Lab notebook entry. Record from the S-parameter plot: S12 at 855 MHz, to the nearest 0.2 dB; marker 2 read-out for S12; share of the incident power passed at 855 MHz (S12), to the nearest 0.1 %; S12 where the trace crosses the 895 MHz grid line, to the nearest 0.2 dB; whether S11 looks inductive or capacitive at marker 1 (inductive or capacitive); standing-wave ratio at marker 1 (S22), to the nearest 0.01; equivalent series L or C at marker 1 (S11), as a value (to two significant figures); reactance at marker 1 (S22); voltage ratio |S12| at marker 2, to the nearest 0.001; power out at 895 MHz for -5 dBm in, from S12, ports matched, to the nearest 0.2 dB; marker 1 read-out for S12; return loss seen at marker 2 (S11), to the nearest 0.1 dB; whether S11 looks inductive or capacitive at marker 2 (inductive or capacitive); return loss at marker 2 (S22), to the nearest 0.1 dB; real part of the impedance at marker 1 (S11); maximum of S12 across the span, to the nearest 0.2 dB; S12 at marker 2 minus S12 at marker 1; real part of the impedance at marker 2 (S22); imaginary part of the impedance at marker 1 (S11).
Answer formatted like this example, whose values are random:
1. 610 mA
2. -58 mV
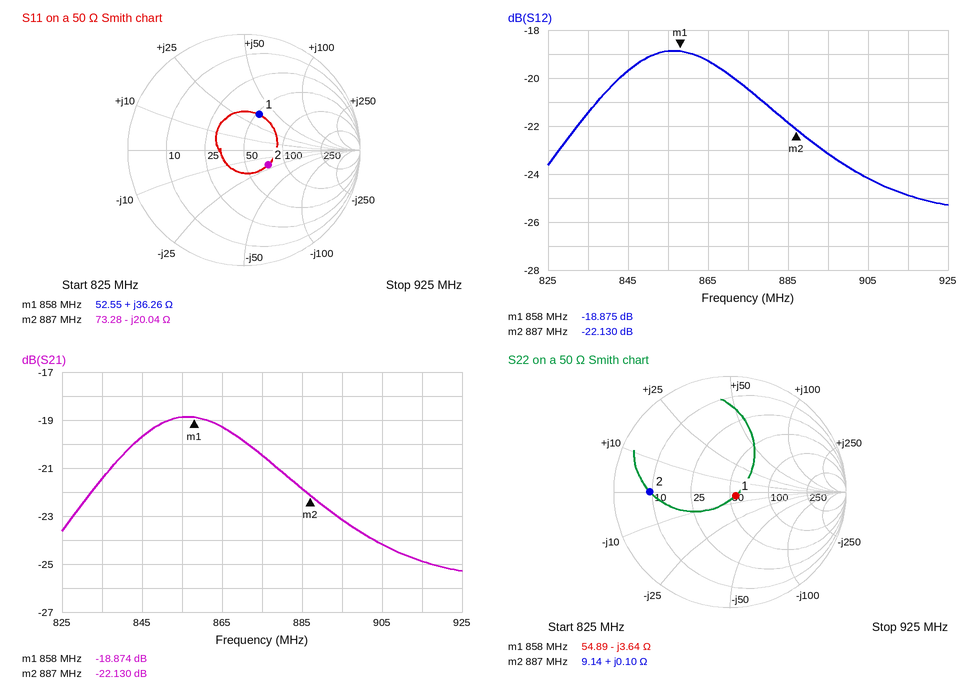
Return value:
1. -18.8 dB
2. -22.130 dB
3. 1.3 %
4. -23.2 dB
5. inductive
6. 1.12
7. 6.7 nH
8. -3.64 Ω
9. 0.078
10. -28.2 dBm
11. -18.875 dB
12. 12.2 dB
13. capacitive
14. 3.2 dB
15. 52.55 Ω
16. -18.8 dB
17. -3.255 dB
18. 9.14 Ω
19. +36.26 Ω
